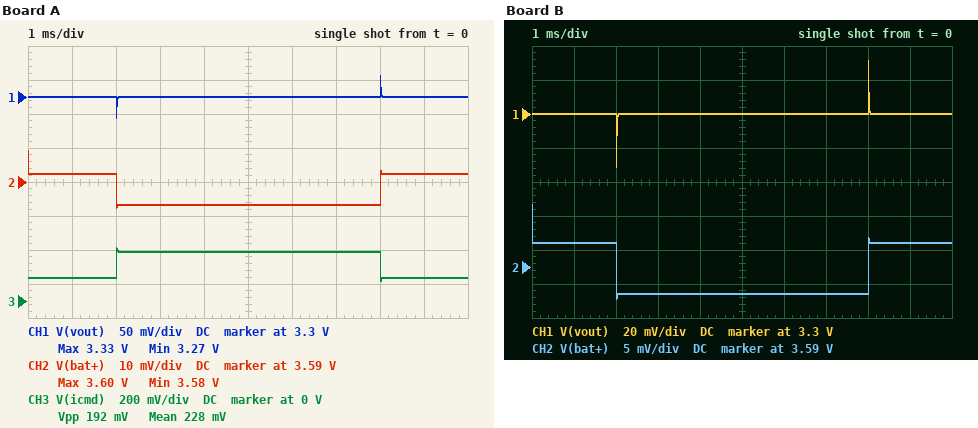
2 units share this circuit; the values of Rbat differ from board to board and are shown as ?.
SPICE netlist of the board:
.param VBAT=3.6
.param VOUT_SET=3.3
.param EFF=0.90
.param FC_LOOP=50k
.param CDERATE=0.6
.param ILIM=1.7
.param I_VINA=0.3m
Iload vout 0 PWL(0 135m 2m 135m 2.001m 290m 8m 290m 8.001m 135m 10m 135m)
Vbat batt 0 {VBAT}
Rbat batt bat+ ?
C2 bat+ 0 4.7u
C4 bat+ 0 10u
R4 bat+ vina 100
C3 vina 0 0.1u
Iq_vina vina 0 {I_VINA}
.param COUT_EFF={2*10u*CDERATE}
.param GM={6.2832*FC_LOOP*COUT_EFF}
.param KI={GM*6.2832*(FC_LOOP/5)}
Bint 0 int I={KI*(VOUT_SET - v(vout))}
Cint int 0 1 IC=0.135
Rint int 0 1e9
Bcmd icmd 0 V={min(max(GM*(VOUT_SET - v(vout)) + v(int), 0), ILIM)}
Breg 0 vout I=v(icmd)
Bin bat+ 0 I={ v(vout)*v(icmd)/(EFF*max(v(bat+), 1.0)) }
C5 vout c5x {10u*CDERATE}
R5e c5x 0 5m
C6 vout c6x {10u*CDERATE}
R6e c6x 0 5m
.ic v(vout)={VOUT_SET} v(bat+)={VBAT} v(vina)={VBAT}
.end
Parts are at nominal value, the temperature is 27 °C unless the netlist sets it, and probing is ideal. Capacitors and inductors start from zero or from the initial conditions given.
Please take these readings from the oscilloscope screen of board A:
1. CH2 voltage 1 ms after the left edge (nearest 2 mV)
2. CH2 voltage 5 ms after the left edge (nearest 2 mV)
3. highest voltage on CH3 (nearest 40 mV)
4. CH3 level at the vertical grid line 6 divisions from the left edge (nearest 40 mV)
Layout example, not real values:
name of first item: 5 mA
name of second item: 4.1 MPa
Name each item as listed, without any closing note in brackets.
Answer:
CH2 voltage 1 ms after the left edge: 3.592 V
CH2 voltage 5 ms after the left edge: 3.584 V
highest voltage on CH3: 320 mV
CH3 level at the vertical grid line 6 divisions from the left edge: 280 mV
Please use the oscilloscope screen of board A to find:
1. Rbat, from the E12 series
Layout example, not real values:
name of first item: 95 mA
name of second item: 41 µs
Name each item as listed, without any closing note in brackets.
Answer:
Rbat, from the E12 series: 0.056 Ω
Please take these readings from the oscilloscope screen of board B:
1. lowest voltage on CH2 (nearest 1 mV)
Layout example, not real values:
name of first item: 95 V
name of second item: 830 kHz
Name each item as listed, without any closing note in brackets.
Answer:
lowest voltage on CH2: 3.585 V
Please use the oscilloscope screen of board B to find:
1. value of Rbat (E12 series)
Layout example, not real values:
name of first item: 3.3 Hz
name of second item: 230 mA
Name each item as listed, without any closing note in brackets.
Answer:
value of Rbat: 0.047 Ω
